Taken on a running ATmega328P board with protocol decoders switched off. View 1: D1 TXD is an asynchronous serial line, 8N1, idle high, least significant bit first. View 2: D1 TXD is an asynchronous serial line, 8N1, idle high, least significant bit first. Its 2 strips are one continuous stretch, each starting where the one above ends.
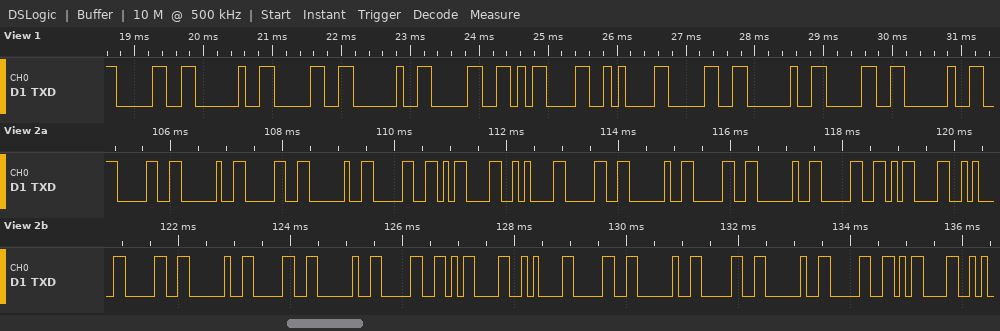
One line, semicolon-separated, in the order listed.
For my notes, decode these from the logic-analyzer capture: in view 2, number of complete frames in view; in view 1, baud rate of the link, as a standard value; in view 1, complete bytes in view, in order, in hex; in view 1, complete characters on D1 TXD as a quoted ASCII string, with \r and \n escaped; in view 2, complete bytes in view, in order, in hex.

27; 9600 baud; 30 20 30 20 30 0D 0A 30 20 30 20; "0 0 0\r\n0 0 "; 30 20 30 20 30 0D 0A 30 20 30 20 30 0D 0A 30 20 30 20 30 0D 0A 30 20 30 20 30 0D
